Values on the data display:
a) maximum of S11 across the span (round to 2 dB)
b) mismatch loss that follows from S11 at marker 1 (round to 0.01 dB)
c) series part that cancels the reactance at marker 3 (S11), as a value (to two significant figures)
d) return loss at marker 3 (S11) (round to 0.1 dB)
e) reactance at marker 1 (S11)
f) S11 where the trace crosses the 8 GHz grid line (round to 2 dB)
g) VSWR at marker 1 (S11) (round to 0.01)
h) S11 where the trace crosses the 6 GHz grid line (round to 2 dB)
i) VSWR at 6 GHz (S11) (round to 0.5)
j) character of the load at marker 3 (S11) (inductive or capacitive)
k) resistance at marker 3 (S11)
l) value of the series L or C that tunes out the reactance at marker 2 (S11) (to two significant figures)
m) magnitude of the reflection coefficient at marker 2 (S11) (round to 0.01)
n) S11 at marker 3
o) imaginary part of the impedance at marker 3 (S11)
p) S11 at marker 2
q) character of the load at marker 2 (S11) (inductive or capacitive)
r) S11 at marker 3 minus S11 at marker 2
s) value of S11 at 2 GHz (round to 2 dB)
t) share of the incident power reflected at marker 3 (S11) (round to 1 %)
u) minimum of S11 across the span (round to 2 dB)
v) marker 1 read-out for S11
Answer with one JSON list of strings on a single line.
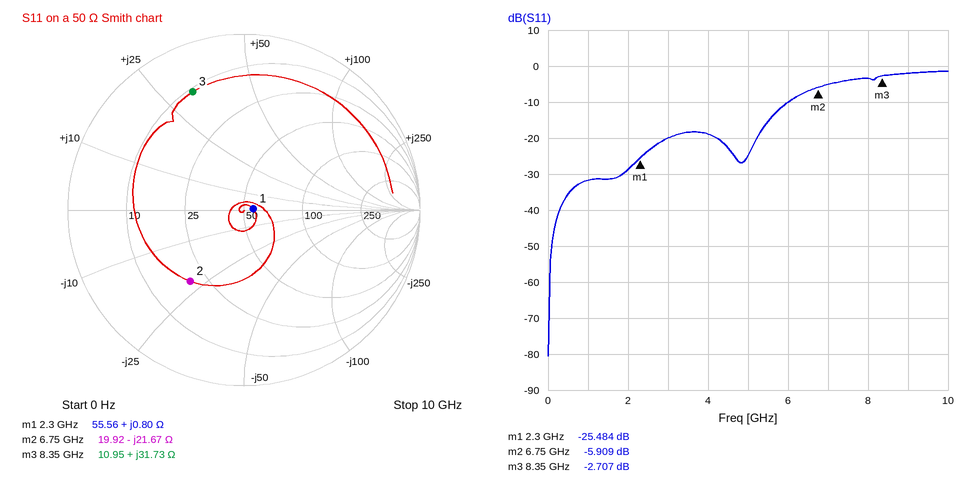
["-2 dB", "0.01 dB", "600 fF", "2.7 dB", "+0.80 Ω", "-4 dB", "1.11", "-10 dB", "2.0", "inductive", "10.95 Ω", "510 pH", "0.51", "-2.707 dB", "+31.73 Ω", "-5.909 dB", "capacitive", "3.202 dB", "-28 dB", "54 %", "-80 dB", "-25.484 dB"]
